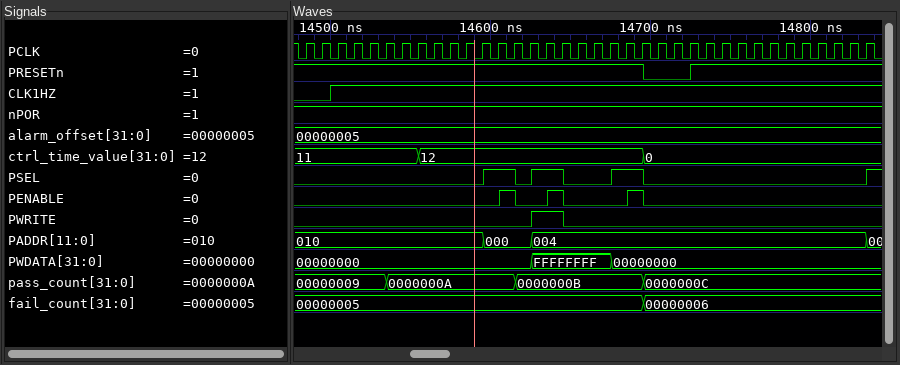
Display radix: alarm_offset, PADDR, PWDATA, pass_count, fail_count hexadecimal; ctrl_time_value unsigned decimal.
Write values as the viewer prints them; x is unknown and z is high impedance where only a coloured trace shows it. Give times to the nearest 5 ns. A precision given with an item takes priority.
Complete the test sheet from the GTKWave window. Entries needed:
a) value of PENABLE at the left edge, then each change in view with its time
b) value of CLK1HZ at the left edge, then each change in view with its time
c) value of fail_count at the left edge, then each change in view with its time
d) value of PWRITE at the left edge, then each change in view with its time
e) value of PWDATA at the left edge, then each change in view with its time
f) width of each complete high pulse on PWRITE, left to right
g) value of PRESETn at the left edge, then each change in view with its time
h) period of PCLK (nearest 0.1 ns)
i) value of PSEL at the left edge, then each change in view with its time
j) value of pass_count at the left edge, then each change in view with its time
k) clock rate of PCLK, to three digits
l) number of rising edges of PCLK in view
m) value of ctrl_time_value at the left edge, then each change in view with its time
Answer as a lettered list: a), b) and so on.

a) 0, 1 at 14605 ns, 0 at 14615 ns, 1 at 14635 ns, 0 at 14645 ns, 1 at 14685 ns, 0 at 14695 ns
b) 0, 1 at 14500 ns
c) 00000005, 00000006 at 14695 ns
d) 0, 1 at 14625 ns, 0 at 14645 ns
e) 00000000, FFFFFFFF at 14625 ns, 00000000 at 14675 ns
f) 20 ns
g) 1, 0 at 14695 ns, 1 at 14725 ns
h) 10 ns
i) 0, 1 at 14595 ns, 0 at 14615 ns, 1 at 14625 ns, 0 at 14645 ns, 1 at 14675 ns, 0 at 14695 ns, 1 at 14835 ns
j) 00000009, 0000000A at 14535 ns, 0000000B at 14615 ns, 0000000C at 14695 ns
k) 100 MHz
l) 36
m) 11, 12 at 14555 ns, 0 at 14695 ns
